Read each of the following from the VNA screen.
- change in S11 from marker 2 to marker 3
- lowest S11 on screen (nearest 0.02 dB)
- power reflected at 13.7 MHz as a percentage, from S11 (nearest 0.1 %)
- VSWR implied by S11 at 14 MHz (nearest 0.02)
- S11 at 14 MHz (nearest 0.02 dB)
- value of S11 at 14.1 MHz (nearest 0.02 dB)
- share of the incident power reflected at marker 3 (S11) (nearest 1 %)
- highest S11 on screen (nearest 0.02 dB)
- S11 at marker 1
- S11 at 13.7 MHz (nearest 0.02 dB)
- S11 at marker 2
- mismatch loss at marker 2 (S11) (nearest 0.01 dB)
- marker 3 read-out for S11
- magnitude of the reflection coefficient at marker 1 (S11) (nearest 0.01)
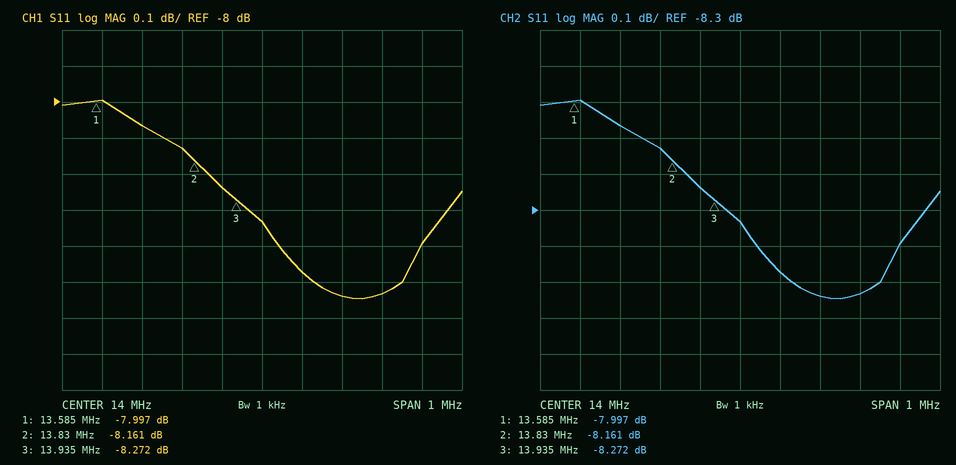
-0.111 dB
-8.54 dB
15.6 %
2.24
-8.34 dB
-8.48 dB
15 %
-8.00 dB
-7.997 dB
-8.06 dB
-8.161 dB
0.72 dB
-8.272 dB
0.40
